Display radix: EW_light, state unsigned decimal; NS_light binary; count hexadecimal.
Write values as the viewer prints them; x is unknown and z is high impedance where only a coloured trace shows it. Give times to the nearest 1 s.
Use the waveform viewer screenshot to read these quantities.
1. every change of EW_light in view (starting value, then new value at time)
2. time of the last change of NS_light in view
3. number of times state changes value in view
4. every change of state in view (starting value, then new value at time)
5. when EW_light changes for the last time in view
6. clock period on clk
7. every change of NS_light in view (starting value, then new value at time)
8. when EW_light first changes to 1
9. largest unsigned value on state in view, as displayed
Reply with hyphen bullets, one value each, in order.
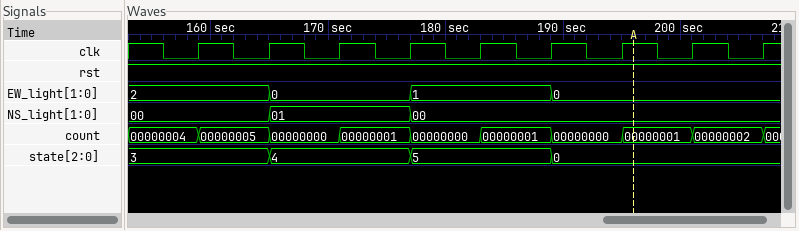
- 2, 0 at 165 s, 1 at 177 s, 0 at 189 s
- 177 s
- 3
- 3, 4 at 165 s, 5 at 177 s, 0 at 189 s
- 189 s
- 6 s
- 00, 01 at 165 s, 00 at 177 s
- 177 s
- 5
